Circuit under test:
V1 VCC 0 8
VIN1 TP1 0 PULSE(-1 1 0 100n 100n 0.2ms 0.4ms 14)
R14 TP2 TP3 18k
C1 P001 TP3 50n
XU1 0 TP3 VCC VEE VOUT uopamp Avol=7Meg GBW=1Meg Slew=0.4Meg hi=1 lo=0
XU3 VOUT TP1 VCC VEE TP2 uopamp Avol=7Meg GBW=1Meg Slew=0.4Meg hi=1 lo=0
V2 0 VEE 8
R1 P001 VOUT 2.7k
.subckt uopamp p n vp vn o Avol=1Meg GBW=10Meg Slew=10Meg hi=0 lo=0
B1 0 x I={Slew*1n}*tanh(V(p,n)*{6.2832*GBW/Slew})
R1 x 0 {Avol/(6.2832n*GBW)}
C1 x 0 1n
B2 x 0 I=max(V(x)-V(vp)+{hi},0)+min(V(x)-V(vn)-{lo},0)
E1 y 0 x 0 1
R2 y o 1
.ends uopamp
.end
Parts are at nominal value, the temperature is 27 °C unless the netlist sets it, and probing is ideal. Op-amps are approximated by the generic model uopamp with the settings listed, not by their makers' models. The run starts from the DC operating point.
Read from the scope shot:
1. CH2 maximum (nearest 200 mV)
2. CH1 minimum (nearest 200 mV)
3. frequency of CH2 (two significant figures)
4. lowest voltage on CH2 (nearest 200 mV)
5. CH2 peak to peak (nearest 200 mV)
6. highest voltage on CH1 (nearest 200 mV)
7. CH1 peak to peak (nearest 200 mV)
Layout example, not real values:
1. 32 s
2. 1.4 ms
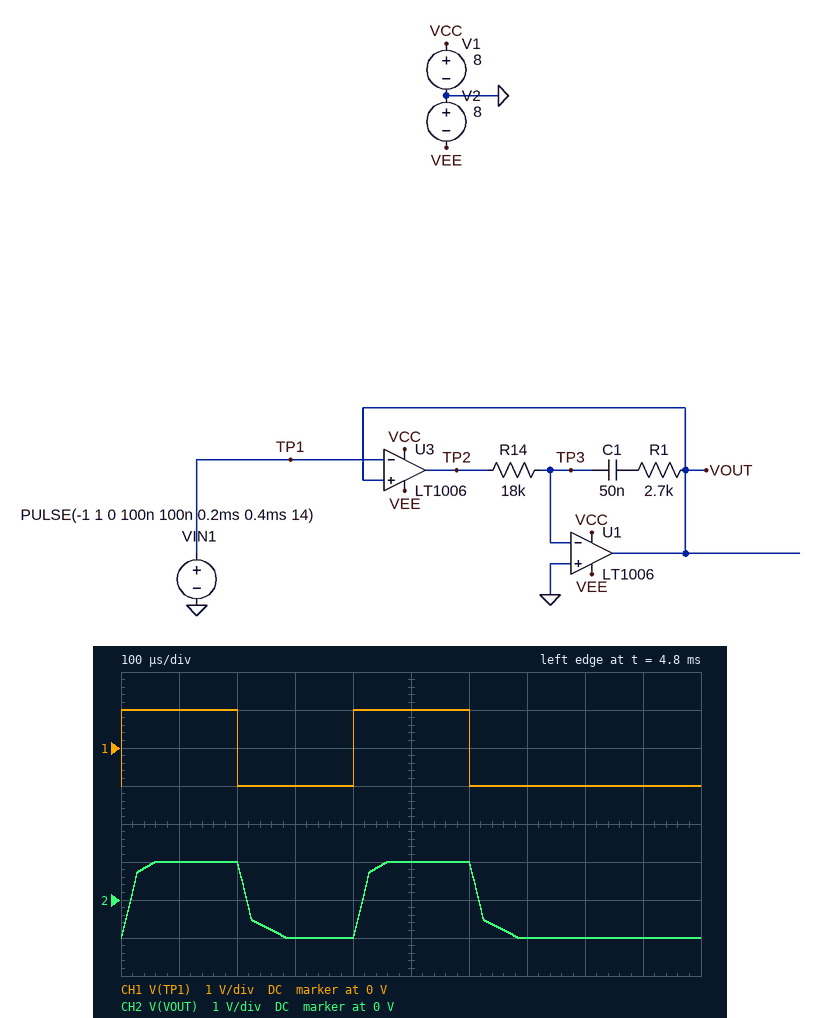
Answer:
1. 1.0 V
2. -1.0 V
3. 2.5 kHz
4. -1.0 V
5. 2.0 V
6. 1.0 V
7. 2.0 V
